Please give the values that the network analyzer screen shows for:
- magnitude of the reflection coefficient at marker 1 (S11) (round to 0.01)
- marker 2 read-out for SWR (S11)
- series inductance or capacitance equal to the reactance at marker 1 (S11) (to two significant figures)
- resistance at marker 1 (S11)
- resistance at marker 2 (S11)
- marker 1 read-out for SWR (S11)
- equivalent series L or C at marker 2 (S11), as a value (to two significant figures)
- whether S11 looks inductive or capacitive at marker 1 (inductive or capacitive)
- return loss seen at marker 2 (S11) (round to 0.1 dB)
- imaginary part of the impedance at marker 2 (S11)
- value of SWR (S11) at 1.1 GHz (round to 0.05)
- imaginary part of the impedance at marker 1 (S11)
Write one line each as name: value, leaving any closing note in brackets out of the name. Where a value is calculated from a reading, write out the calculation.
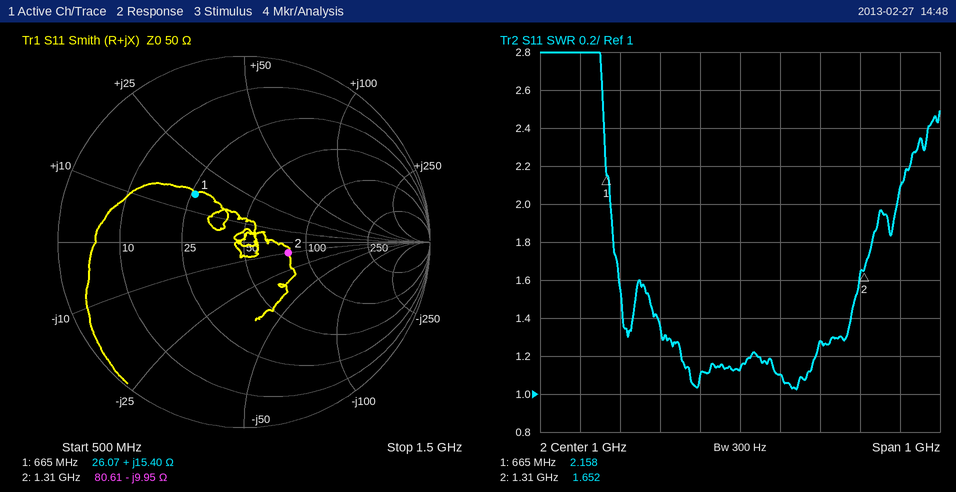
magnitude of the reflection coefficient at marker 1 (S11): 0.37
marker 2 read-out for SWR: 1.652
series inductance or capacitance equal to the reactance at marker 1 (S11): L = 15.4 Ω/(2π × 665 MHz) ≈ 3.7 nH
resistance at marker 1: 26.07 Ω
resistance at marker 2: 80.61 Ω
marker 1 read-out for SWR: 2.158
equivalent series L or C at marker 2 (S11), as a value: C = 1/(2π × 1.31 GHz × 9.95 Ω) ≈ 12 pF
whether S11 looks inductive or capacitive at marker 1: inductive
return loss seen at marker 2 (S11): 12.2 dB
imaginary part of the impedance at marker 2: -9.95 Ω
value of SWR (S11) at 1.1 GHz: 1.10
imaginary part of the impedance at marker 1: +15.40 Ω
